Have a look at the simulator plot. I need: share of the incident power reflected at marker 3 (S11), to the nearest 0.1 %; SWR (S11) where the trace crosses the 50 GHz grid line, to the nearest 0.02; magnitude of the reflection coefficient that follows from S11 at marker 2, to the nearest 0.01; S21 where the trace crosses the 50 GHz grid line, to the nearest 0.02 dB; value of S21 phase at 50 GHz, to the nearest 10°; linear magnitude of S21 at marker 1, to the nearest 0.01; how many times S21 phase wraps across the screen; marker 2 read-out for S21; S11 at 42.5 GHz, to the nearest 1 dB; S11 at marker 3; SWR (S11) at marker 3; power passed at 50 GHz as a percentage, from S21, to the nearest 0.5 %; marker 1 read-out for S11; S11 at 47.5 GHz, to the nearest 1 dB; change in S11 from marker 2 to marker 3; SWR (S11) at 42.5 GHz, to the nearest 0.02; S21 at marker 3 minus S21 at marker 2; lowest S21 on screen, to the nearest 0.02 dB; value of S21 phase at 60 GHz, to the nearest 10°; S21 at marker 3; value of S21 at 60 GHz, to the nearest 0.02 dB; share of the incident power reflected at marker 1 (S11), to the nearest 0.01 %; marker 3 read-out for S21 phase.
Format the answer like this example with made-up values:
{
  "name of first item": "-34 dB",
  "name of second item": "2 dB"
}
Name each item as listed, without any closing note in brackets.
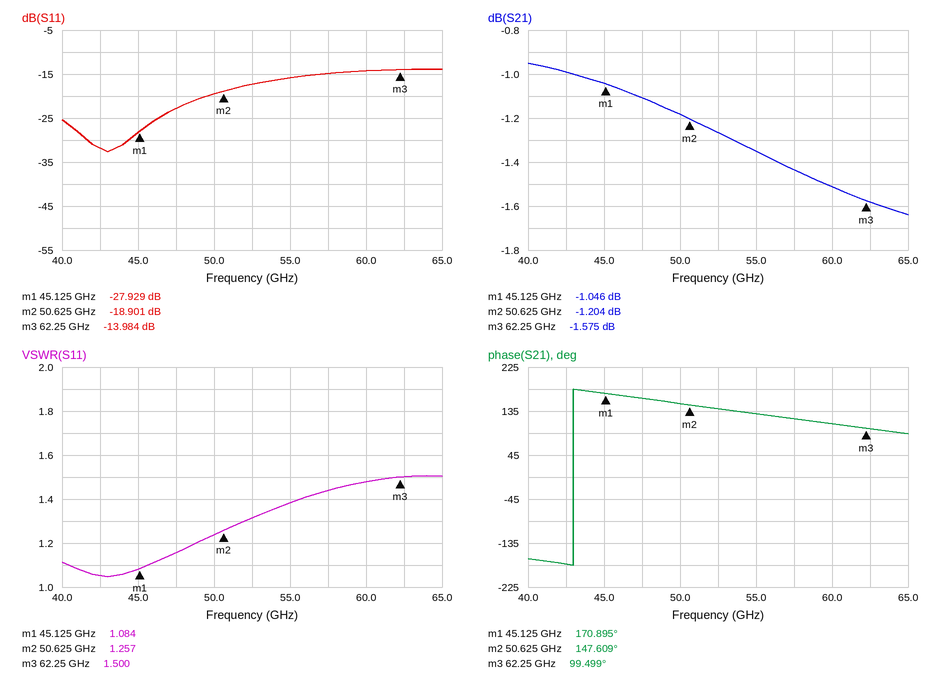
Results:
{
  "share of the incident power reflected at marker 3 (S11), to the nearest 0.1 %": "4.0 %",
  "SWR (S11) where the trace crosses the 50 GHz grid line, to the nearest 0.02": "1.24",
  "magnitude of the reflection coefficient that follows from S11 at marker 2, to the nearest 0.01": "0.11",
  "S21 where the trace crosses the 50 GHz grid line, to the nearest 0.02 dB": "-1.18 dB",
  "value of S21 phase at 50 GHz, to the nearest 10°": "150°",
  "linear magnitude of S21 at marker 1, to the nearest 0.01": "0.89",
  "how many times S21 phase wraps across the screen": "1",
  "marker 2 read-out for S21": "-1.204 dB",
  "S11 at 42.5 GHz, to the nearest 1 dB": "-32 dB",
  "S11 at marker 3": "-13.984 dB",
  "SWR (S11) at marker 3": "1.500",
  "power passed at 50 GHz as a percentage, from S21, to the nearest 0.5 %": "76.0 %",
  "marker 1 read-out for S11": "-27.929 dB",
  "S11 at 47.5 GHz, to the nearest 1 dB": "-23 dB",
  "change in S11 from marker 2 to marker 3": "4.917 dB",
  "SWR (S11) at 42.5 GHz, to the nearest 0.02": "1.06",
  "S21 at marker 3 minus S21 at marker 2": "-0.371 dB",
  "lowest S21 on screen, to the nearest 0.02 dB": "-1.64 dB",
  "value of S21 phase at 60 GHz, to the nearest 10°": "110°",
  "S21 at marker 3": "-1.575 dB",
  "value of S21 at 60 GHz, to the nearest 0.02 dB": "-1.52 dB",
  "share of the incident power reflected at marker 1 (S11), to the nearest 0.01 %": "0.16 %",
  "marker 3 read-out for S21 phase": "99.499°"
}
